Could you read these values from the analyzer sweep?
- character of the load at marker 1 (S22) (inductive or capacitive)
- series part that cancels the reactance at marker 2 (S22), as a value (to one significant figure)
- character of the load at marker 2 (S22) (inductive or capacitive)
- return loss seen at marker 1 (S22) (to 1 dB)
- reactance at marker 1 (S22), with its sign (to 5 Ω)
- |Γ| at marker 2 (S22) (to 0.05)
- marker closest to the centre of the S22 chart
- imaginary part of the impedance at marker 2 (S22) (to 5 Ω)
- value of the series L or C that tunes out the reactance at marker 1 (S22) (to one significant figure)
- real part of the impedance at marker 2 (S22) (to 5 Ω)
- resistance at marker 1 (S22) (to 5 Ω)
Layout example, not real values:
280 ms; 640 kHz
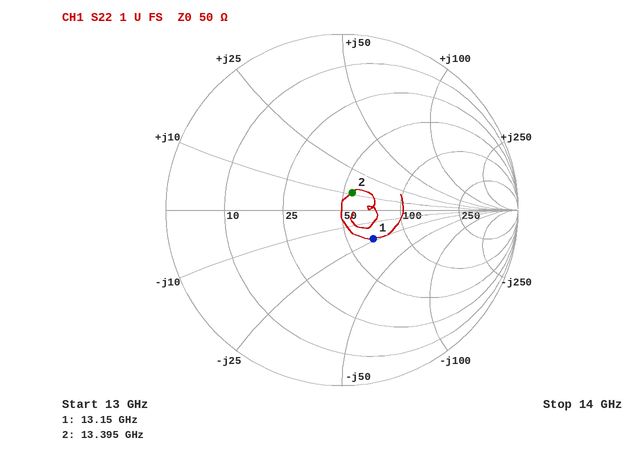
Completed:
capacitive; 1 pF; inductive; 12 dB; -25 Ω; 0.10; marker 2; +10 Ω; 300 pH; 55 Ω; 65 Ω
